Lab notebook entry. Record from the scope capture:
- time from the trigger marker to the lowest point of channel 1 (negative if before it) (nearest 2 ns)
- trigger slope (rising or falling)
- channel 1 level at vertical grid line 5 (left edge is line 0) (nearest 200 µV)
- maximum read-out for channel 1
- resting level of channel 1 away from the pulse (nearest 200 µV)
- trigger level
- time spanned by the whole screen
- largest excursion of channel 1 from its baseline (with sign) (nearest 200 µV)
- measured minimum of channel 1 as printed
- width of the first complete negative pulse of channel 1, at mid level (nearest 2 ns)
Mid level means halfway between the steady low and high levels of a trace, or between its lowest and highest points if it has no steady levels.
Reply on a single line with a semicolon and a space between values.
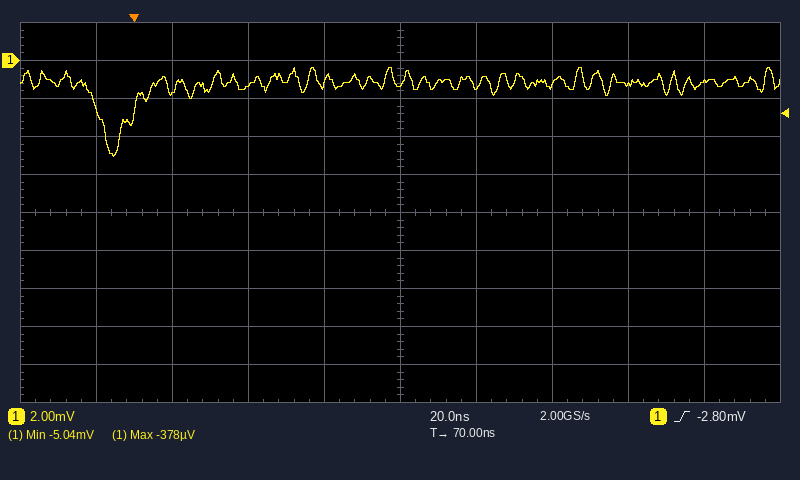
-6 ns; rising; -1.2 mV; -378 µV; -1.2 mV; -2.80 mV; 200 ns; -3.8 mV; -5.04 mV; 10 ns
